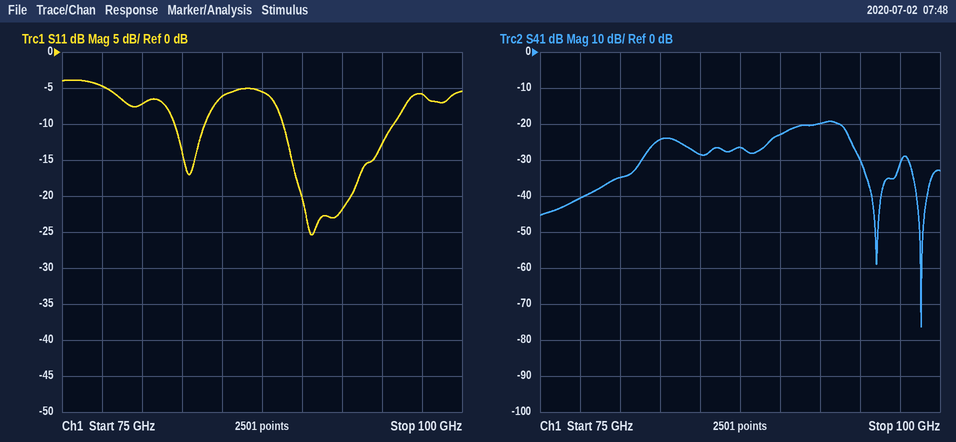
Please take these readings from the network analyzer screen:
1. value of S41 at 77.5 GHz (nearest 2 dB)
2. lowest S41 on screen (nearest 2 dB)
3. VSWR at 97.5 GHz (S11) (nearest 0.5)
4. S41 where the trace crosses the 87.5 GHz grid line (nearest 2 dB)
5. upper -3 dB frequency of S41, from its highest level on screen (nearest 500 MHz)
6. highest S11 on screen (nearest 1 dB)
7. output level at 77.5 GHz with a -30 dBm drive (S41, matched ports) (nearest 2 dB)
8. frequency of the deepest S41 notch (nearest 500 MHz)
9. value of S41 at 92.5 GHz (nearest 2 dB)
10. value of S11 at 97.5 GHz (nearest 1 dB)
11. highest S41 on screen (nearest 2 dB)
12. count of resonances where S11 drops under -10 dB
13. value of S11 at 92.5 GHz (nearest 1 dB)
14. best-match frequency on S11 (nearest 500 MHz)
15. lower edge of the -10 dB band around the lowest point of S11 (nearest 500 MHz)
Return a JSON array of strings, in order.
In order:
["-40 dB", "-76 dB", "3.0", "-26 dB", "94.0 GHz", "-4 dB", "-70 dBm", "99.0 GHz", "-20 dB", "-6 dB", "-20 dB", "2", "-22 dB", "90.5 GHz", "89.0 GHz"]
